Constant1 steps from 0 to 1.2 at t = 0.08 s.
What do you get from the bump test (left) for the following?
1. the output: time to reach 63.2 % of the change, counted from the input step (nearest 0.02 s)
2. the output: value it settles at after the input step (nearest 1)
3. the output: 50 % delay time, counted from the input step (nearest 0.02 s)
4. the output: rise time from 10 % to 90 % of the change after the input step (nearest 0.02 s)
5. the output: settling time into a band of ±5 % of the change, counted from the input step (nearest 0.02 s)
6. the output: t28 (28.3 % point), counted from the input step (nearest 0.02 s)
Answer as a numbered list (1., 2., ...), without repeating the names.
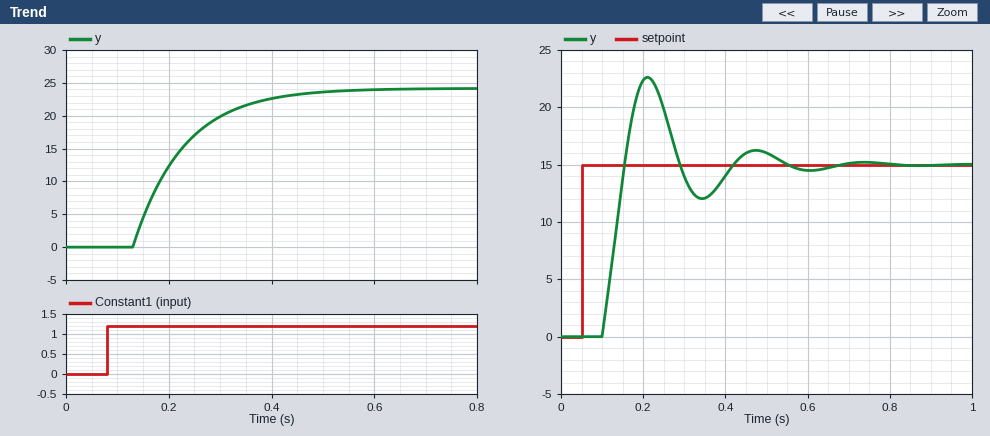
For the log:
1. 0.14 s
2. 24
3. 0.12 s
4. 0.22 s
5. 0.34 s
6. 0.08 s
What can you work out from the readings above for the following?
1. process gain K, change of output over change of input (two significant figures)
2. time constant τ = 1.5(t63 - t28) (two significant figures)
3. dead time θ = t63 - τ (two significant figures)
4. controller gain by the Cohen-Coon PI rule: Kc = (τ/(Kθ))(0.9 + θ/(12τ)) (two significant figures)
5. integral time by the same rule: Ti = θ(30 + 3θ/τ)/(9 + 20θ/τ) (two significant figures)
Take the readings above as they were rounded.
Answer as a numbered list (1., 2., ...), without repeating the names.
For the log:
1. 20
2. 0.090 s
3. 0.050 s
4. 0.085
5. 0.079 s
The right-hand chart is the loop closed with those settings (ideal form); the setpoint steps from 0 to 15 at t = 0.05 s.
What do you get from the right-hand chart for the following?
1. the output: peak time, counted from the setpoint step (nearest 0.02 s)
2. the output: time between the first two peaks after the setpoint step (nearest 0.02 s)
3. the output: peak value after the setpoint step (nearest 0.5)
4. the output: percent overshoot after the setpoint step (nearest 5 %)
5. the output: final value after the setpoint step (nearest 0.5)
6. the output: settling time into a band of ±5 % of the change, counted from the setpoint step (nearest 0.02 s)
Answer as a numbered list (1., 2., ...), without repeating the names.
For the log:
1. 0.16 s
2. 0.26 s
3. 22.5
4. 50 %
5. 15.0
6. 0.46 s
